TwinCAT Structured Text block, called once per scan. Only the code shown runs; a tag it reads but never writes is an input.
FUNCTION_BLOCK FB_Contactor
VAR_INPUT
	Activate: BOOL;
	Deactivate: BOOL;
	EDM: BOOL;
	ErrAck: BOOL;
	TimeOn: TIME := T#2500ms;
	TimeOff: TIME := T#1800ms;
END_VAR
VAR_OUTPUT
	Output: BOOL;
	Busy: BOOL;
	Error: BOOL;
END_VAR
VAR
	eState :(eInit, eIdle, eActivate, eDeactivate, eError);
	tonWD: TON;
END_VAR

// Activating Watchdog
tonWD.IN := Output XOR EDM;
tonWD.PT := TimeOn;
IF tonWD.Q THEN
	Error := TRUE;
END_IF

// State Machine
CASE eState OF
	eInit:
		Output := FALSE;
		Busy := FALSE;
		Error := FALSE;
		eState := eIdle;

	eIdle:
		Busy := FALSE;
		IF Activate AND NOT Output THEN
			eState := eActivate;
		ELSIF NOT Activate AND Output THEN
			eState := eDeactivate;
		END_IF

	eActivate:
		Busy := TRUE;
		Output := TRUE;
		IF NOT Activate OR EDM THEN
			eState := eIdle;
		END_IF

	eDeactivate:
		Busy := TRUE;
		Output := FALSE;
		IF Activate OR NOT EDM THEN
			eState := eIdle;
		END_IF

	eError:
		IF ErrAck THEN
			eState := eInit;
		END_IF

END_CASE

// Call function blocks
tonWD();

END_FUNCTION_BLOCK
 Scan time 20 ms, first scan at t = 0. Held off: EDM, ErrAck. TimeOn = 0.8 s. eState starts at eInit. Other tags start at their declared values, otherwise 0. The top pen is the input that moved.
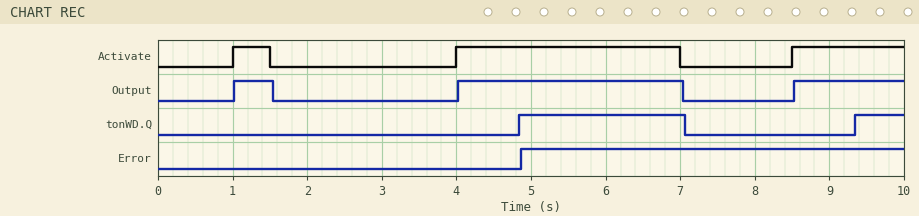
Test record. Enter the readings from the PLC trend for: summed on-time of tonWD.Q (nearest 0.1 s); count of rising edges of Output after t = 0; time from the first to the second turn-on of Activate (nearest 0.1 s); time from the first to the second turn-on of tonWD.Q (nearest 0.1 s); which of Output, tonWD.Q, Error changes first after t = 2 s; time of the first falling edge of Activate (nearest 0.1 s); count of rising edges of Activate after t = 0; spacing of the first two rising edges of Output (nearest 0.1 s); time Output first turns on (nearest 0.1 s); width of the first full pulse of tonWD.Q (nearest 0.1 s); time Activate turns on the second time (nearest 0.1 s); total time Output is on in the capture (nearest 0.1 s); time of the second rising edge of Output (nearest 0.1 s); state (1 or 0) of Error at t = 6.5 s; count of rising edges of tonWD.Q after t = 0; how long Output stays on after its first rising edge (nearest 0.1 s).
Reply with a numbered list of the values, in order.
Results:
1. 2.9 s
2. 3
3. 3.0 s
4. 4.5 s
5. Output
6. 1.5 s
7. 3
8. 3.0 s
9. 1.0 s
10. 2.2 s
11. 4.0 s
12. 5.0 s
13. 4.0 s
14. 1
15. 2
16. 0.5 s
